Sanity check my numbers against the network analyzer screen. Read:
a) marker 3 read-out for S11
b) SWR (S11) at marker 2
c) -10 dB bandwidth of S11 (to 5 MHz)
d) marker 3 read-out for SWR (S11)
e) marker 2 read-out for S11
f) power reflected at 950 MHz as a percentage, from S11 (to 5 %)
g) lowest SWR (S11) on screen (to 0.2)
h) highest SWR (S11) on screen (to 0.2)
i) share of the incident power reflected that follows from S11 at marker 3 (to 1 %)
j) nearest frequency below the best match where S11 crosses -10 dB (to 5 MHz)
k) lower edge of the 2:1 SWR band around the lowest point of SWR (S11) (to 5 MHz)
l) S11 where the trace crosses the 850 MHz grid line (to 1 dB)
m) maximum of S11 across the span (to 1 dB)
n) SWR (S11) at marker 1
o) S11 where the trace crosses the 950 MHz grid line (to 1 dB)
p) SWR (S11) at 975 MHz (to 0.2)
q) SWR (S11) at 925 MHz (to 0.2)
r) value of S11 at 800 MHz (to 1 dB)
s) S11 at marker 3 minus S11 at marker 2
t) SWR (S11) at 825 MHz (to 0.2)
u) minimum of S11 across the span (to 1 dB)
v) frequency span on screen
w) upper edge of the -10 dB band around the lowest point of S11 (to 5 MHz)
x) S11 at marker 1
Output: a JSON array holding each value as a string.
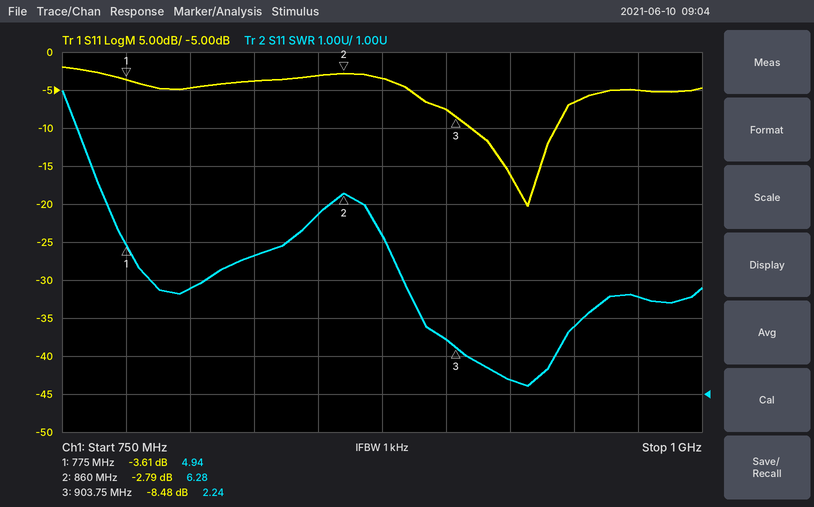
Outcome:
["-8.48 dB", "6.28", "35 MHz", "2.24", "-2.79 dB", "20 %", "1.2", "9.0", "14 %", "910 MHz", "910 MHz", "-3 dB", "-2 dB", "4.94", "-7 dB", "3.6", "1.4", "-5 dB", "-5.69 dB", "4.6", "-20 dB", "250 MHz", "945 MHz", "-3.61 dB"]
